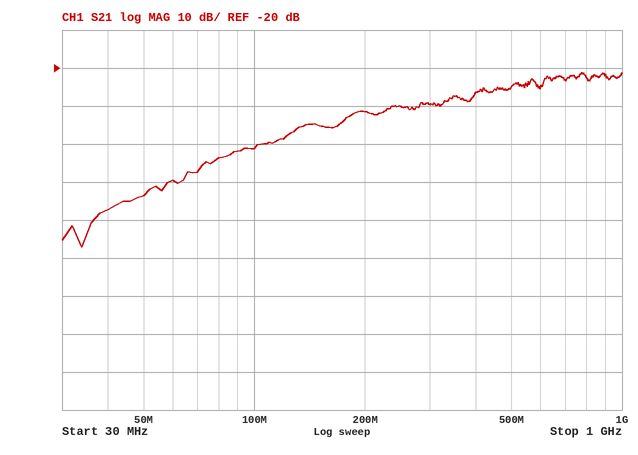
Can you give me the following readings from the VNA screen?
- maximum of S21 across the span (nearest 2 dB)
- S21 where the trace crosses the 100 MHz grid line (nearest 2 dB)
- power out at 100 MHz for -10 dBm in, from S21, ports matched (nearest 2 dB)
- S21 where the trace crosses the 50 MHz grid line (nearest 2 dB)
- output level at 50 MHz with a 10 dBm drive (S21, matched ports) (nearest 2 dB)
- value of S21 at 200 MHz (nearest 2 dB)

-22 dB
-42 dB
-52 dBm
-54 dB
-44 dBm
-32 dB
